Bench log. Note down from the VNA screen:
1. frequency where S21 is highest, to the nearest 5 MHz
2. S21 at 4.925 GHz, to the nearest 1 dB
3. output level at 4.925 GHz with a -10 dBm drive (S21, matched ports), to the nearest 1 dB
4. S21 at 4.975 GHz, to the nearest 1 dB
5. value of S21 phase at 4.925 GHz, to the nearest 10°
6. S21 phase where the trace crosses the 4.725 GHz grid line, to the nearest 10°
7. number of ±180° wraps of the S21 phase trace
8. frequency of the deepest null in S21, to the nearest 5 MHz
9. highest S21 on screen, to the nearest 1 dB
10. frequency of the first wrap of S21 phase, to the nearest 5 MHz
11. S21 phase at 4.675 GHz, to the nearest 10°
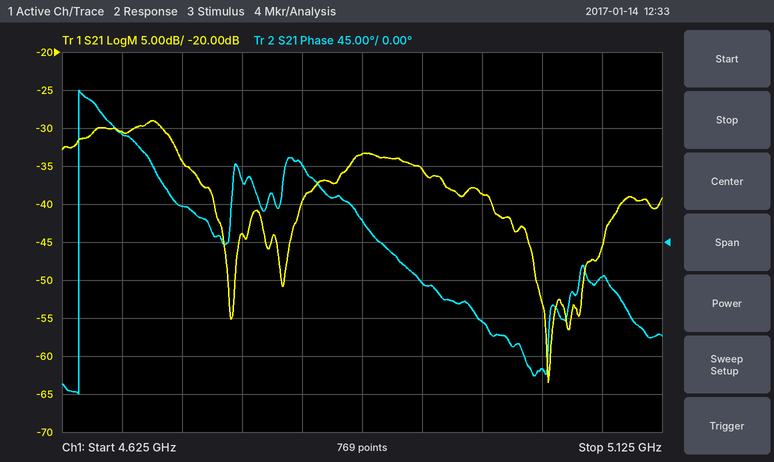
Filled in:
4.700 GHz
-35 dB
-45 dBm
-39 dB
-50°
40°
1
5.030 GHz
-29 dB
4.640 GHz
130°
